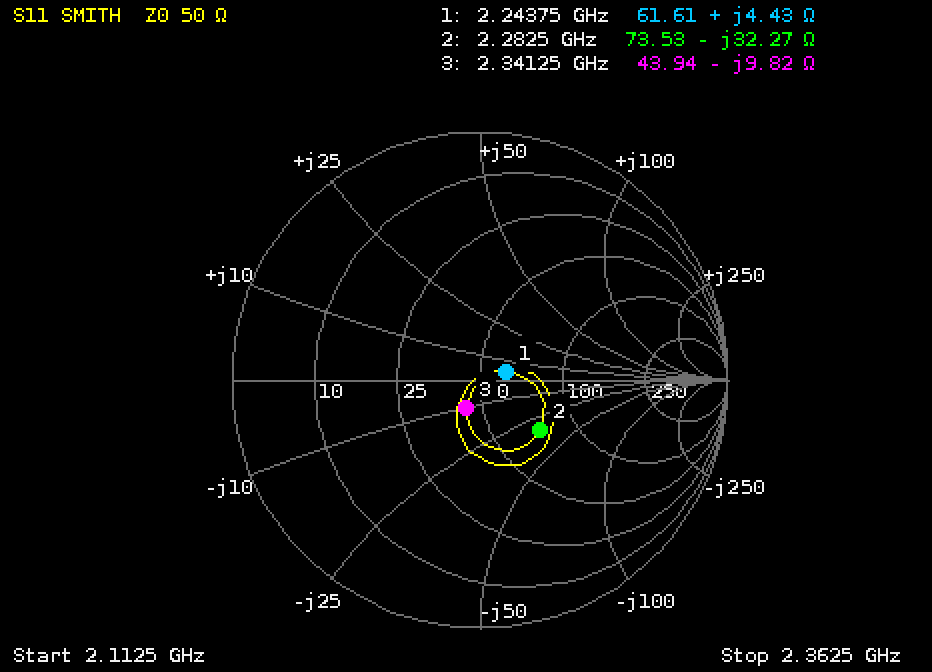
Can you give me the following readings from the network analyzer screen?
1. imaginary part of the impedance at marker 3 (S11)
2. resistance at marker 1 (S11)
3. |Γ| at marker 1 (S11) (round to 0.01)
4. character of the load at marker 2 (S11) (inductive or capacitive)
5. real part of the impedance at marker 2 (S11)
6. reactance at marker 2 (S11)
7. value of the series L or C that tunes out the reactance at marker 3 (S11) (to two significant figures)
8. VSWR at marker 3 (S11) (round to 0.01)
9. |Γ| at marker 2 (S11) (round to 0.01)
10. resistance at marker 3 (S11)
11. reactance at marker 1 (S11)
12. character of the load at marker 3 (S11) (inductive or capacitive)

-9.82 Ω
61.61 Ω
0.11
capacitive
73.53 Ω
-32.27 Ω
670 pH
1.28
0.31
43.94 Ω
+4.43 Ω
capacitive
